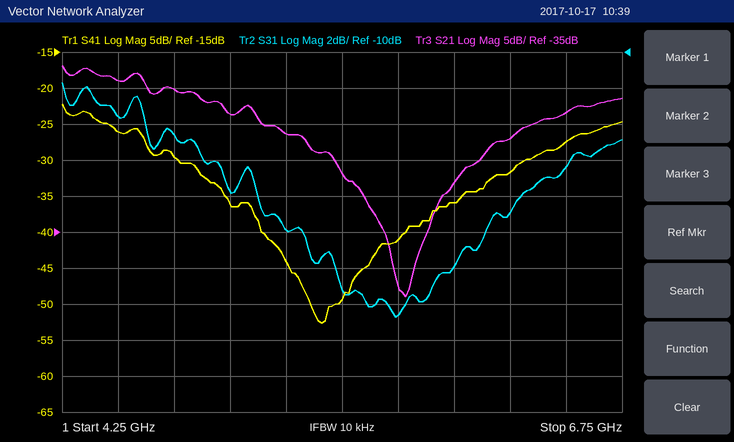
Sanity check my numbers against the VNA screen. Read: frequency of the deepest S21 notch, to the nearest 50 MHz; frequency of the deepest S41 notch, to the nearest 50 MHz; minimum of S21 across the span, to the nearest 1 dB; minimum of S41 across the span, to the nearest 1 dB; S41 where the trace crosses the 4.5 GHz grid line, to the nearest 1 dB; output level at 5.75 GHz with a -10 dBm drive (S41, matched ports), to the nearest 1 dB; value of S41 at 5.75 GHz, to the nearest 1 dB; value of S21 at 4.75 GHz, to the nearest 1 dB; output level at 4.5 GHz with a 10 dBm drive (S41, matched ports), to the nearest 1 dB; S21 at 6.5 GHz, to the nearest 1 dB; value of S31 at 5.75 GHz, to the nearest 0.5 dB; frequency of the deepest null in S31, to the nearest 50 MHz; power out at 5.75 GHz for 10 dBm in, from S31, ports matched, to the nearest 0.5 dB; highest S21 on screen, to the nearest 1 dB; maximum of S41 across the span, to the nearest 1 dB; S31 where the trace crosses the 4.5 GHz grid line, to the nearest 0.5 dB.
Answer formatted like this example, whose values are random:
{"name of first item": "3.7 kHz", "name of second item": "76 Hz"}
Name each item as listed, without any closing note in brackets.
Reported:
{"frequency of the deepest S21 notch, to the nearest 50 MHz": "5.80 GHz", "frequency of the deepest S41 notch, to the nearest 50 MHz": "5.40 GHz", "minimum of S21 across the span, to the nearest 1 dB": "-44 dB", "minimum of S41 across the span, to the nearest 1 dB": "-53 dB", "S41 where the trace crosses the 4.5 GHz grid line, to the nearest 1 dB": "-26 dB", "output level at 5.75 GHz with a -10 dBm drive (S41, matched ports), to the nearest 1 dB": "-51 dBm", "value of S41 at 5.75 GHz, to the nearest 1 dB": "-41 dB", "value of S21 at 4.75 GHz, to the nearest 1 dB": "-15 dB", "output level at 4.5 GHz with a 10 dBm drive (S41, matched ports), to the nearest 1 dB": "-16 dBm", "S21 at 6.5 GHz, to the nearest 1 dB": "-18 dB", "value of S31 at 5.75 GHz, to the nearest 0.5 dB": "-24.5 dB", "frequency of the deepest null in S31, to the nearest 50 MHz": "5.75 GHz", "power out at 5.75 GHz for 10 dBm in, from S31, ports matched, to the nearest 0.5 dB": "-14.5 dBm", "highest S21 on screen, to the nearest 1 dB": "-12 dB", "maximum of S41 across the span, to the nearest 1 dB": "-22 dB", "S31 where the trace crosses the 4.5 GHz grid line, to the nearest 0.5 dB": "-13.5 dB"}
